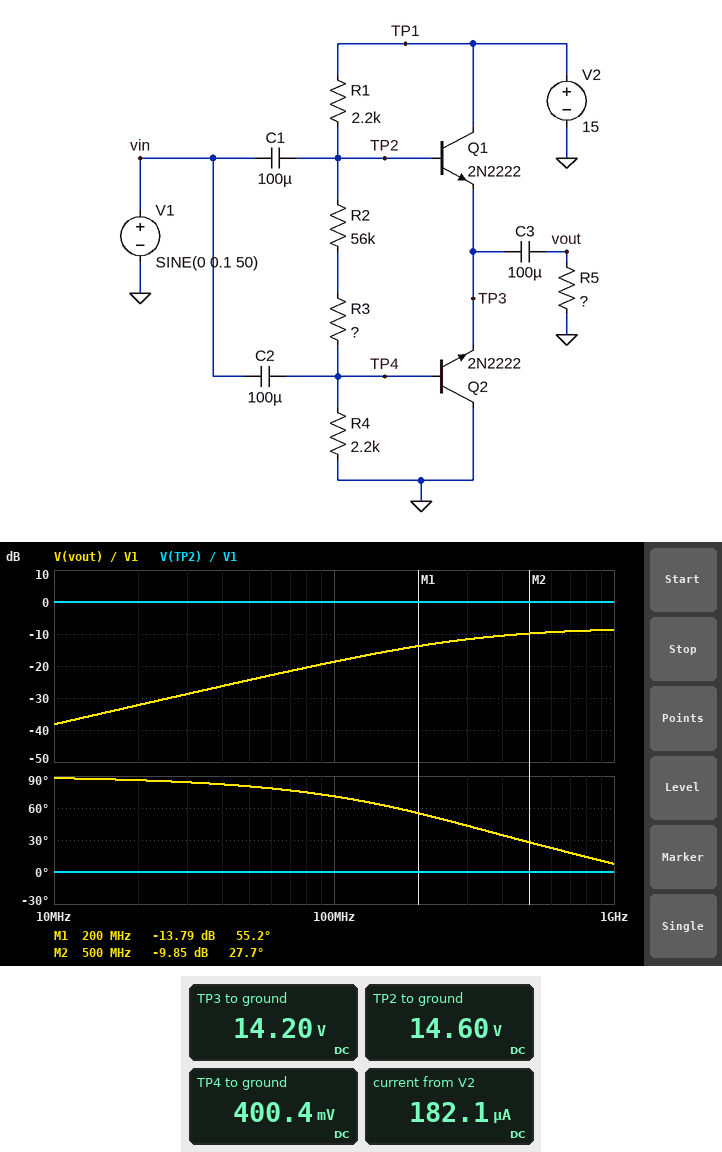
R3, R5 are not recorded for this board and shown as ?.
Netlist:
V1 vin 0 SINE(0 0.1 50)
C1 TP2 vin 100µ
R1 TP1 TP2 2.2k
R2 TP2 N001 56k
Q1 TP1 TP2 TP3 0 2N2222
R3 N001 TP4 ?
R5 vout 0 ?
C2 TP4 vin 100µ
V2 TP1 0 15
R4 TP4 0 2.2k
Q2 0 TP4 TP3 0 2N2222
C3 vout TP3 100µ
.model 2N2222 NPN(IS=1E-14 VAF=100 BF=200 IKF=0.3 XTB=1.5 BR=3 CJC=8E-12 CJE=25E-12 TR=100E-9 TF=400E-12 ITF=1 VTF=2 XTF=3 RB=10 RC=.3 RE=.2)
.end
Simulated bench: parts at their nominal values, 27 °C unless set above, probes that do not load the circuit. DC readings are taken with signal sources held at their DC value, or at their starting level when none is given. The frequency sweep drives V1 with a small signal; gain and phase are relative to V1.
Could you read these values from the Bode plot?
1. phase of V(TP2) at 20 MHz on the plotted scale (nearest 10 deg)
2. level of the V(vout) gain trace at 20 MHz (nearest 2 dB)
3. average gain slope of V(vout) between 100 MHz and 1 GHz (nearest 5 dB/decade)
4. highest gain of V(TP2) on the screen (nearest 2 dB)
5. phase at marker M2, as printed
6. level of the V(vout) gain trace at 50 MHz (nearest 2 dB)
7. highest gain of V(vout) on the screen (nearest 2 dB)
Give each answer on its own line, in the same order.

0 deg
-32 dB
10 dB/decade
0 dB
27.7 deg
-24 dB
-8 dB
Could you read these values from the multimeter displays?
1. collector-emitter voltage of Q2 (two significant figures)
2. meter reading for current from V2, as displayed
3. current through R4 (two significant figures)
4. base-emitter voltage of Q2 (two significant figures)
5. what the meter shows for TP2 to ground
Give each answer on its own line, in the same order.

-14 V
182.1 µA
180 µA
-14 V
14.60 V
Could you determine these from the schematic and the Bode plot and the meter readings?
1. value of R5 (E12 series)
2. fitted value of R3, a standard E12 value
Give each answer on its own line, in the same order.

4.7 Ω
22 kΩ
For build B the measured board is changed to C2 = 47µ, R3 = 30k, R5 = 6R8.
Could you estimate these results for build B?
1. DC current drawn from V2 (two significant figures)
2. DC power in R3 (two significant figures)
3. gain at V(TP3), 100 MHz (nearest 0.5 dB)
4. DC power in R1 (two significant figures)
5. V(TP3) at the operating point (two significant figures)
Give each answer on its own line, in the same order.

170 µA
830 µW
-16.0 dB
61 µW
14 V
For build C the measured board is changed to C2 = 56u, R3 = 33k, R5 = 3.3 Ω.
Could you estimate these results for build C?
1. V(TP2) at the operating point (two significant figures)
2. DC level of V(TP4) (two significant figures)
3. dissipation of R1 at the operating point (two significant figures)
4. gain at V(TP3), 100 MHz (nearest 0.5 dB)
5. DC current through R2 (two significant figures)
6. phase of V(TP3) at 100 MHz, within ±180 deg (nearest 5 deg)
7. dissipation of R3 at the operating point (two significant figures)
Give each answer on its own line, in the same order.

15 V
350 mV
57 µW
-22.0 dB
160 µA
75 deg
850 µW
